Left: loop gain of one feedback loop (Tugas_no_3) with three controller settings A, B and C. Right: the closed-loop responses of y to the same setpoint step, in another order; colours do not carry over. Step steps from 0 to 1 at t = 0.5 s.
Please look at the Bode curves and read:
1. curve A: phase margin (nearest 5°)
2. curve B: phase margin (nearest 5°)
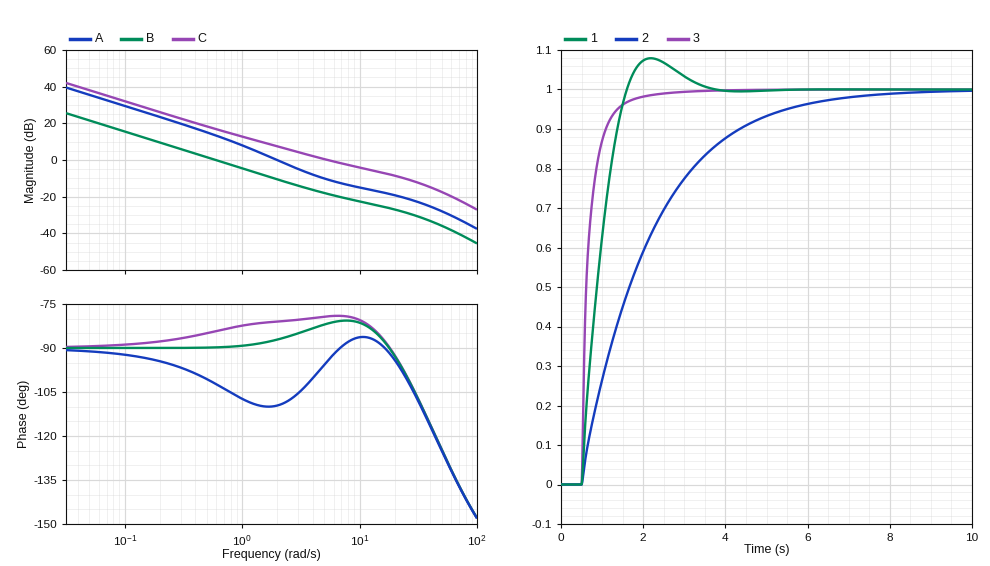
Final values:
70°
90°
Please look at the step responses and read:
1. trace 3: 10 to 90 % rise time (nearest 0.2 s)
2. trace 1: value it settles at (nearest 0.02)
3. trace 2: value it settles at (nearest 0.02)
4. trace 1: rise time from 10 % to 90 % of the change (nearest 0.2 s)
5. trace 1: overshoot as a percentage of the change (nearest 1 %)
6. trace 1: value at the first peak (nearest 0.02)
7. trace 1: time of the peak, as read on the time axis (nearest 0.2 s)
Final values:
0.6 s
1.00
1.00
0.8 s
8 %
1.08
2.2 s
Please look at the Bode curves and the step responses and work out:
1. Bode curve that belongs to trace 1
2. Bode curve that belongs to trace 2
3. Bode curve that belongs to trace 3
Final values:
A
B
C
